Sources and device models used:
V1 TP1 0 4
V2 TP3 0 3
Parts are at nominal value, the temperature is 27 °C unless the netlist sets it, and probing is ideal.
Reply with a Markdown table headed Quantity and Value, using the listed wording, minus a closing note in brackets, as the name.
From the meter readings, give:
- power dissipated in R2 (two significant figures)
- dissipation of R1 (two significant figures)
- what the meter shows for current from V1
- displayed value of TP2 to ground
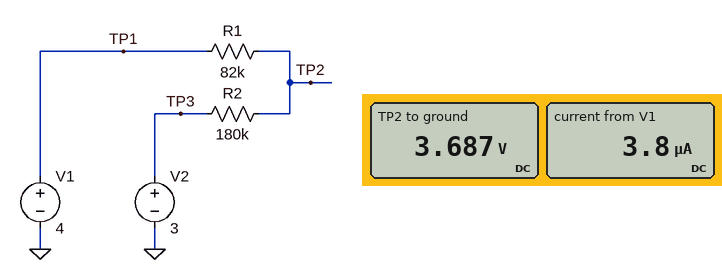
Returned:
| Quantity | Value |
|---|---|
| power dissipated in R2 | 2.6 µW |
| dissipation of R1 | 1.2 µW |
| what the meter shows for current from V1 | 3.8 µA |
| displayed value of TP2 to ground | 3.687 V |
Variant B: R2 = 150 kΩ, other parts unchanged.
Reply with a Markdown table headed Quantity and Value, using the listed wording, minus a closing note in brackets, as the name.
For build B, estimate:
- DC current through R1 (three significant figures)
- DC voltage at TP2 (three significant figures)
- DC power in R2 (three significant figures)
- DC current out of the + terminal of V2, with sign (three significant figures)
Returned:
| Quantity | Value |
|---|---|
| DC current through R1 | 4.31 µA |
| DC voltage at TP2 | 3.65 V |
| DC power in R2 | 2.79 µW |
| DC current out of the + terminal of V2, with sign | -4.31 µA |
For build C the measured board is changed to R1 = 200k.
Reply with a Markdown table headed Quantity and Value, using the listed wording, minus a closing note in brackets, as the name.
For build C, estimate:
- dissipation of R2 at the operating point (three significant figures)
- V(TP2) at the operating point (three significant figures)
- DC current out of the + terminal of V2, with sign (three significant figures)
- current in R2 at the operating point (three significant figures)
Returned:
| Quantity | Value |
|---|---|
| dissipation of R2 at the operating point | 1.25 µW |
| V(TP2) at the operating point | 3.47 V |
| DC current out of the + terminal of V2, with sign | -2.63 µA |
| current in R2 at the operating point | 2.63 µA |
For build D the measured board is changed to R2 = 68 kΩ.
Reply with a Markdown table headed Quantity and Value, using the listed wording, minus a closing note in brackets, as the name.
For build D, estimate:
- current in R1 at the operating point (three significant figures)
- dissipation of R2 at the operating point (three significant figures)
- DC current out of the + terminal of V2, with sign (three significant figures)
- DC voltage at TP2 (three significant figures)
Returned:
| Quantity | Value |
|---|---|
| current in R1 at the operating point | 6.67 µA |
| dissipation of R2 at the operating point | 3.02 µW |
| DC current out of the + terminal of V2, with sign | -6.67 µA |
| DC voltage at TP2 | 3.45 V |
